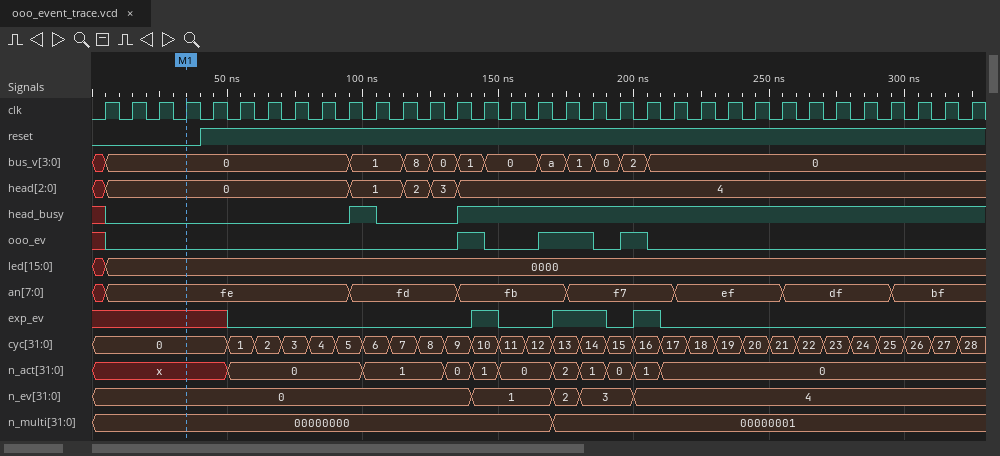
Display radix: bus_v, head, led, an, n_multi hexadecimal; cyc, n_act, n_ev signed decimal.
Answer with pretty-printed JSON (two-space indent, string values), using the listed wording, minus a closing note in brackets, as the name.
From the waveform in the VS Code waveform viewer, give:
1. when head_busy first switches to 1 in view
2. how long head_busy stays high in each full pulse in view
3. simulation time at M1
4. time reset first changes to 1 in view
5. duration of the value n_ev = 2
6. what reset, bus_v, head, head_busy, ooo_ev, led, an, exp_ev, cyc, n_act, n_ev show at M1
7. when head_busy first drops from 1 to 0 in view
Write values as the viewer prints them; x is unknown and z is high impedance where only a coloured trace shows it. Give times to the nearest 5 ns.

{
  "when head_busy first switches to 1 in view": "95 ns",
  "how long head_busy stays high in each full pulse in view": "10 ns",
  "simulation time at M1": "35 ns",
  "time reset first changes to 1 in view": "40 ns",
  "duration of the value n_ev = 2": "10 ns",
  "what reset, bus_v, head, head_busy, ooo_ev, led, an, exp_ev, cyc, n_act, n_ev show at M1": "reset=0, bus_v=0, head=0, head_busy=0, ooo_ev=0, led=0000, an=fe, exp_ev=x, cyc=0, n_act=x, n_ev=0",
  "when head_busy first drops from 1 to 0 in view": "105 ns"
}
